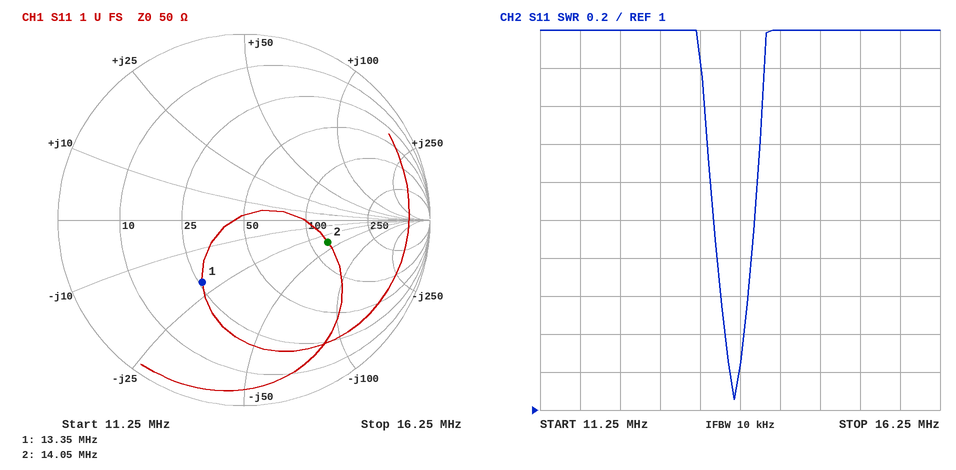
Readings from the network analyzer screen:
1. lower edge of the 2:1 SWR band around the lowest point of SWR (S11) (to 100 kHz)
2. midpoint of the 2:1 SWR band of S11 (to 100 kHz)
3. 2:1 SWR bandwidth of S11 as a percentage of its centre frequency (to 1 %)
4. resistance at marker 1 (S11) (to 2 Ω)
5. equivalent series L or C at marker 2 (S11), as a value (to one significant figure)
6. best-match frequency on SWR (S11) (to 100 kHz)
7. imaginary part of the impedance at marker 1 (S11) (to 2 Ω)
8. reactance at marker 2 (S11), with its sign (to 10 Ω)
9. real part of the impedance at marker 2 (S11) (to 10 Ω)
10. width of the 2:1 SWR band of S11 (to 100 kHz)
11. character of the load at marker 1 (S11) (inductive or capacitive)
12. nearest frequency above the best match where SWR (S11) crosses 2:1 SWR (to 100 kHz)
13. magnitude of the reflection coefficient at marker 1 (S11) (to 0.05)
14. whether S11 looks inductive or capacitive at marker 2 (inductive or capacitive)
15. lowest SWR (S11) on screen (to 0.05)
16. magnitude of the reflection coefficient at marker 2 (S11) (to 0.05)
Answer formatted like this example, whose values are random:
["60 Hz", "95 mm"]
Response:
["13.4 MHz", "13.7 MHz", "4 %", "26 Ω", "300 pF", "13.7 MHz", "-20 Ω", "-40 Ω", "120 Ω", "500 kHz", "capacitive", "13.9 MHz", "0.40", "capacitive", "1.05", "0.45"]
